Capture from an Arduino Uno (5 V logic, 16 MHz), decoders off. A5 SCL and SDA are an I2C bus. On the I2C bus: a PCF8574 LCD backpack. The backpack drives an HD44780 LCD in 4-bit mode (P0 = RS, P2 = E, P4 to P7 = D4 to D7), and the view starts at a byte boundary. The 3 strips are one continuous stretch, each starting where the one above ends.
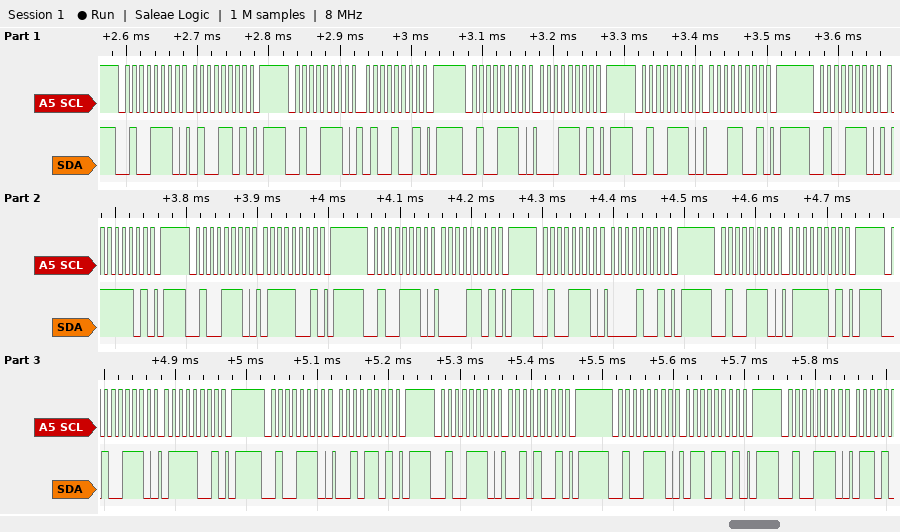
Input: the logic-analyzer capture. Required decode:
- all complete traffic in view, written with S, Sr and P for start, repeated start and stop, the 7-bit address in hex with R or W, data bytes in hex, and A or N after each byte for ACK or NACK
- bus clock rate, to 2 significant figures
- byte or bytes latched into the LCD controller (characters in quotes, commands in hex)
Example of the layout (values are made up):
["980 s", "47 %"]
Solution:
["S 27W A 4D A P S 27W A 49 A P S 27W A 1D A P S 27W A 19 A P S 27W A 7D A P S 27W A 79 A P S 27W A 0D A P S 27W A 09 A P S 27W A 7D A P S 27W A 79 A P S 27W A 2D A P S 27W A 29 A P S 27W A 6D A P S 27W A", "100 kHz", "'A' 'p' 'r'"]
